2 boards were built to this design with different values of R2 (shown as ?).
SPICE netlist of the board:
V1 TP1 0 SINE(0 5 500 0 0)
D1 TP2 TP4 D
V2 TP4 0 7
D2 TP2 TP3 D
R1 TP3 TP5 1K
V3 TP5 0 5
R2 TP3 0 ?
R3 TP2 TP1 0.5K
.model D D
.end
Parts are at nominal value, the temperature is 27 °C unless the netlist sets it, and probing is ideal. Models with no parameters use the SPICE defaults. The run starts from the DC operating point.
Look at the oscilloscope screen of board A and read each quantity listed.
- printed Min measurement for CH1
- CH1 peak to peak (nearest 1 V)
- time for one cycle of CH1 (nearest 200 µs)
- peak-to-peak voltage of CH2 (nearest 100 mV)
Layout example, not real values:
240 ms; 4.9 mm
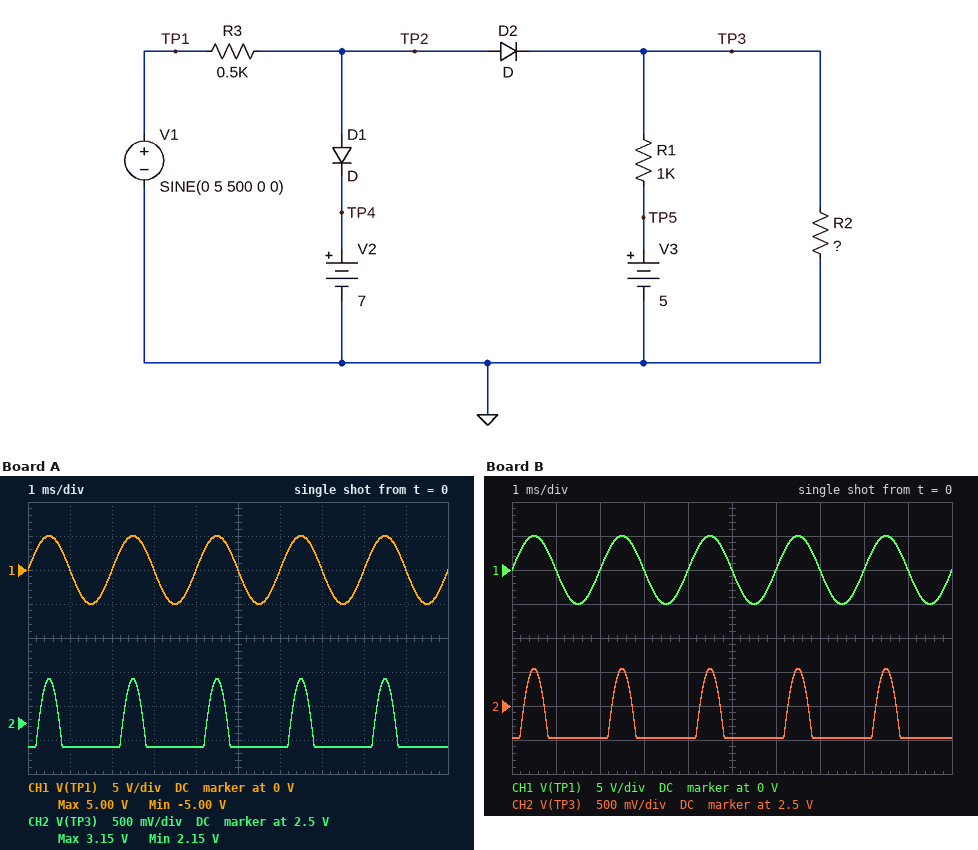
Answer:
-5.00 V; 10 V; 2.0 ms; 1.0 V
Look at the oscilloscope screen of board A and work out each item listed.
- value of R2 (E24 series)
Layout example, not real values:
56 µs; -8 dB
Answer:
750 Ω
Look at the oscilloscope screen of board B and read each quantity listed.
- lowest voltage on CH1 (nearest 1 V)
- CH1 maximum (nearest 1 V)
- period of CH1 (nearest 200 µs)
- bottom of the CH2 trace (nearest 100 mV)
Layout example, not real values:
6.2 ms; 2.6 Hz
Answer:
-5 V; 5 V; 2.0 ms; 2.0 V
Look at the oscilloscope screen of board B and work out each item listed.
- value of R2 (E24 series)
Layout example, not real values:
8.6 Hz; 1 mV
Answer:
680 Ω
